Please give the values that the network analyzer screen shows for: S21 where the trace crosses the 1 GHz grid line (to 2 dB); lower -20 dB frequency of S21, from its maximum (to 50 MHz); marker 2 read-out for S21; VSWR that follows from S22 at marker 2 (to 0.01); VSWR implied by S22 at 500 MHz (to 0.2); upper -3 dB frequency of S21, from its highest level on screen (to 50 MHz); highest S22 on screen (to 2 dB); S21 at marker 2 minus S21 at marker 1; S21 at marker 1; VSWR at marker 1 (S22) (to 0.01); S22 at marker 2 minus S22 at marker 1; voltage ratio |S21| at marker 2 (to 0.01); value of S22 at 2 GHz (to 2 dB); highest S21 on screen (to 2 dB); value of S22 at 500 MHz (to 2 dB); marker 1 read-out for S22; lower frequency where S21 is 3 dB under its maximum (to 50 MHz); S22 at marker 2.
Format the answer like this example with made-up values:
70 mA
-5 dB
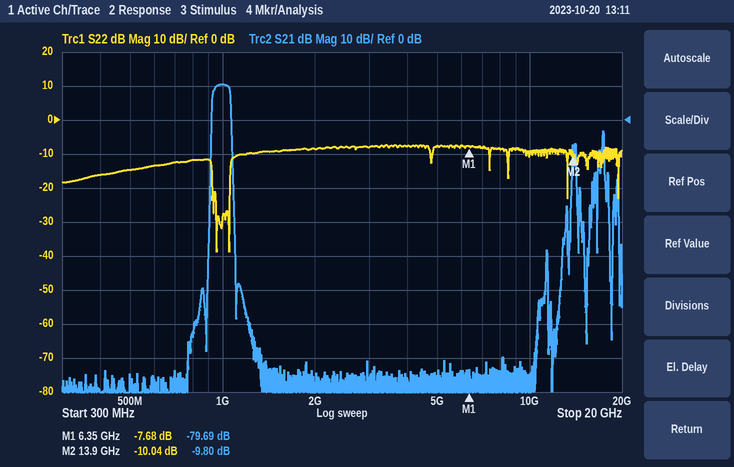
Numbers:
10 dB
900 MHz
-9.80 dB
1.92
1.4
1.05 GHz
-8 dB
69.89 dB
-79.69 dB
2.41
-2.36 dB
0.32
-8 dB
10 dB
-14 dB
-7.68 dB
950 MHz
-10.04 dB
